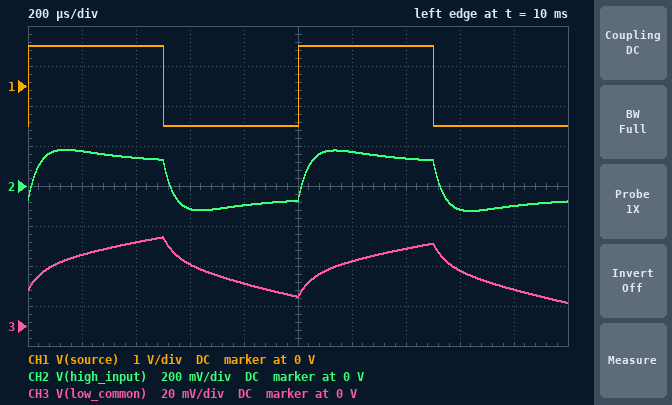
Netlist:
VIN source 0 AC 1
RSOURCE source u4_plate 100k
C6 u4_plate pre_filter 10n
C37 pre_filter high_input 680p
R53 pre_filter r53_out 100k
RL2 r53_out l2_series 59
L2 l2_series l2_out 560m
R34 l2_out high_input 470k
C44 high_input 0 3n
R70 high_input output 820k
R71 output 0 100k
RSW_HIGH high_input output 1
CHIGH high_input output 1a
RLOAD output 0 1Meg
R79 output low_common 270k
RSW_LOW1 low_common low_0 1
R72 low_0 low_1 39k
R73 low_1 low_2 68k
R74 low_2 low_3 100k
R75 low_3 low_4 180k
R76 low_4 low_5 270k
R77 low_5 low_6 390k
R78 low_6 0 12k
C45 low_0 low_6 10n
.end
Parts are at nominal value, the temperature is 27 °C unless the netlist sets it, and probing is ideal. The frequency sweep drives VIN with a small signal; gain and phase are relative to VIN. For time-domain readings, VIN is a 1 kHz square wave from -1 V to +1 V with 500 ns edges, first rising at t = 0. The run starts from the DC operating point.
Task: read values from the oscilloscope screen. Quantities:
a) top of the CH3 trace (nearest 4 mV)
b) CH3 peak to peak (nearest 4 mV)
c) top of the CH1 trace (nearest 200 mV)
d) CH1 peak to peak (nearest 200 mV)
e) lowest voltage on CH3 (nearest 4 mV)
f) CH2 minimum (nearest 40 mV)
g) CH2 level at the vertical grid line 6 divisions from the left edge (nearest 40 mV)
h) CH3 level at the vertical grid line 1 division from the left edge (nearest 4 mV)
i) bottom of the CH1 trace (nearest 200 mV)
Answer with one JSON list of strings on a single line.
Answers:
["44 mV", "32 mV", "1.0 V", "2.0 V", "12 mV", "-120 mV", "160 mV", "36 mV", "-1.0 V"]
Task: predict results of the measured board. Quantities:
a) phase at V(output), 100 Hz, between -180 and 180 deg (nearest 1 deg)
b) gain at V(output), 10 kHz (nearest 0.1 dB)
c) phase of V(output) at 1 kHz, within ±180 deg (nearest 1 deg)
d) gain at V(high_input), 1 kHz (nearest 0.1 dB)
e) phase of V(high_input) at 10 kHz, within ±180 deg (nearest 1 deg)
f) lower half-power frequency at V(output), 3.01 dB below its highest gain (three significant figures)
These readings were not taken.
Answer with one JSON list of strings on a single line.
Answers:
["10 deg", "-26.0 dB", "-2 deg", "-17.8 dB", "-69 deg", "49.4 Hz"]
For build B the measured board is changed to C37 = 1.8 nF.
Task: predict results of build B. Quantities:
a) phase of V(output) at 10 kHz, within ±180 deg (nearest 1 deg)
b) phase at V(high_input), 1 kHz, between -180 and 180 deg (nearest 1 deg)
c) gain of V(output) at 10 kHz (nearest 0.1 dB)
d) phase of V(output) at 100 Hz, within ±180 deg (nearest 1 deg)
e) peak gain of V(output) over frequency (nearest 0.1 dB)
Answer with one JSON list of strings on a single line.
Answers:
["-77 deg", "-8 deg", "-25.7 dB", "24 deg", "-13.3 dB"]
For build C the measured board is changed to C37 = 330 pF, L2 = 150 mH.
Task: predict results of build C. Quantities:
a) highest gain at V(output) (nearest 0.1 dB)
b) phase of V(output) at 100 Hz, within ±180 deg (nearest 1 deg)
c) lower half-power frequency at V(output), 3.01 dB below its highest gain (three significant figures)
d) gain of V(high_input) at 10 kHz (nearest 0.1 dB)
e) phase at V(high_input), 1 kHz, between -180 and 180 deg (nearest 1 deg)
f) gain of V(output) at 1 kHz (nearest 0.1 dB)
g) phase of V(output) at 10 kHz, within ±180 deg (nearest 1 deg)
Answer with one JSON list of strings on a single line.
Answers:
["-20.5 dB", "5 deg", "16.0 Hz", "-27.0 dB", "-10 deg", "-21.4 dB", "-58 deg"]
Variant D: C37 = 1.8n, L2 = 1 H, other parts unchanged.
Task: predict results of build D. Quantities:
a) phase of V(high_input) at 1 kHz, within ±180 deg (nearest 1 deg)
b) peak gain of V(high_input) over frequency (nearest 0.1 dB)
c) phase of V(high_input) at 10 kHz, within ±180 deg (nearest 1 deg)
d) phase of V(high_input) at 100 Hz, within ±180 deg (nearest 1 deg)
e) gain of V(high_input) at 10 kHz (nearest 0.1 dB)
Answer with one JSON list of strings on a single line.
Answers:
["-8 deg", "-13.3 dB", "-77 deg", "24 deg", "-25.7 dB"]
